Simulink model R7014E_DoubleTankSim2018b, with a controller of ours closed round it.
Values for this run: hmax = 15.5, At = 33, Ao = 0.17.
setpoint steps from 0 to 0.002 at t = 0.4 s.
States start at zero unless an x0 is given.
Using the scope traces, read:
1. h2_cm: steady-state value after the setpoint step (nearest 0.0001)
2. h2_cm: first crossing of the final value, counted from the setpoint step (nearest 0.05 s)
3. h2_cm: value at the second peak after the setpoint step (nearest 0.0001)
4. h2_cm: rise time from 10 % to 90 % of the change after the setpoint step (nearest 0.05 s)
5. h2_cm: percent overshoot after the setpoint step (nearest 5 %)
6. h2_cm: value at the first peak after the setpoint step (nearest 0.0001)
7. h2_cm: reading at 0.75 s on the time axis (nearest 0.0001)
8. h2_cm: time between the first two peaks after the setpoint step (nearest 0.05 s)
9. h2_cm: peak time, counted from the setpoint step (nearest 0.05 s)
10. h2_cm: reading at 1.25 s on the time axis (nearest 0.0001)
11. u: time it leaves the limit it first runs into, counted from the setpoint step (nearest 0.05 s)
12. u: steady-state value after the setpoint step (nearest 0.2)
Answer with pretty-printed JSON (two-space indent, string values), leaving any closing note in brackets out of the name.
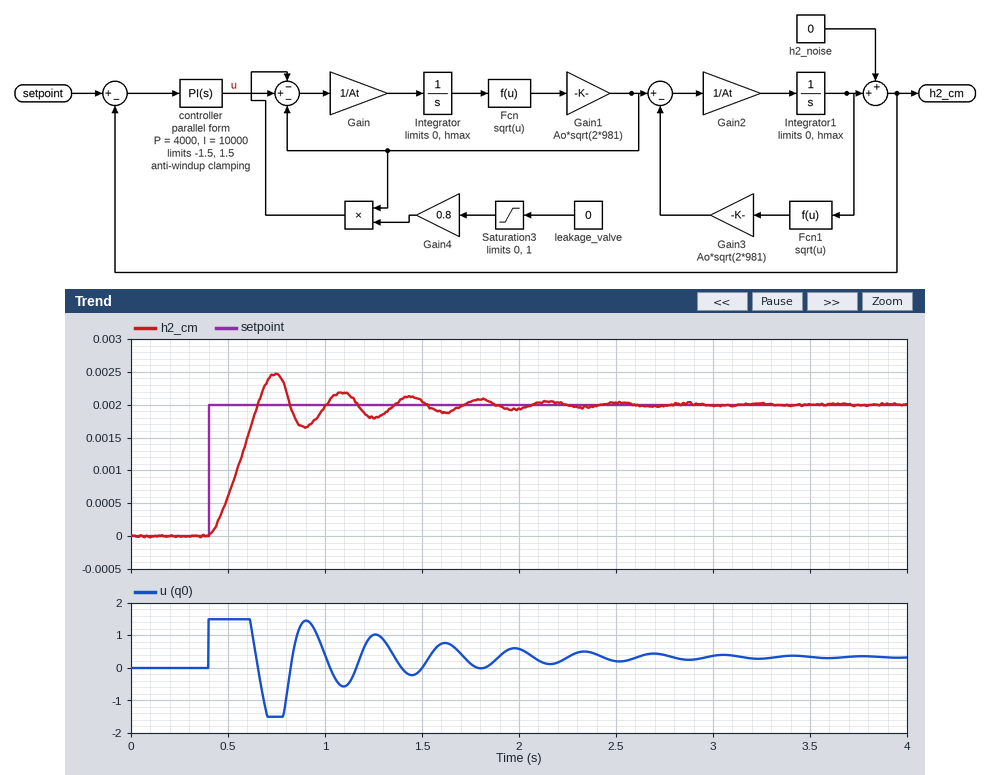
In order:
{
  "h2_cm: steady-state value after the setpoint step": "0.0020",
  "h2_cm: first crossing of the final value, counted from the setpoint step": "0.25 s",
  "h2_cm: value at the second peak after the setpoint step": "0.0022",
  "h2_cm: rise time from 10 % to 90 % of the change after the setpoint step": "0.20 s",
  "h2_cm: percent overshoot after the setpoint step": "25 %",
  "h2_cm: value at the first peak after the setpoint step": "0.0025",
  "h2_cm: reading at 0.75 s on the time axis": "0.0025",
  "h2_cm: time between the first two peaks after the setpoint step": "0.35 s",
  "h2_cm: peak time, counted from the setpoint step": "0.35 s",
  "h2_cm: reading at 1.25 s on the time axis": "0.0018",
  "u: time it leaves the limit it first runs into, counted from the setpoint step": "0.20 s",
  "u: steady-state value after the setpoint step": "0.4"
}
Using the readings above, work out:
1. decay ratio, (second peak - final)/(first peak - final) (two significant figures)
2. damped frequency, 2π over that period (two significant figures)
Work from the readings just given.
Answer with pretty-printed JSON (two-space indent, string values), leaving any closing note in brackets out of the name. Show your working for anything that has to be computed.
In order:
{
  "decay ratio, (second peak - final)/(first peak - final)": "(0.0022 - 0.002) / (0.0025 - 0.002) = 0.40",
  "damped frequency, 2π over that period": "2π / 0.35 = 18 rad/s"
}
